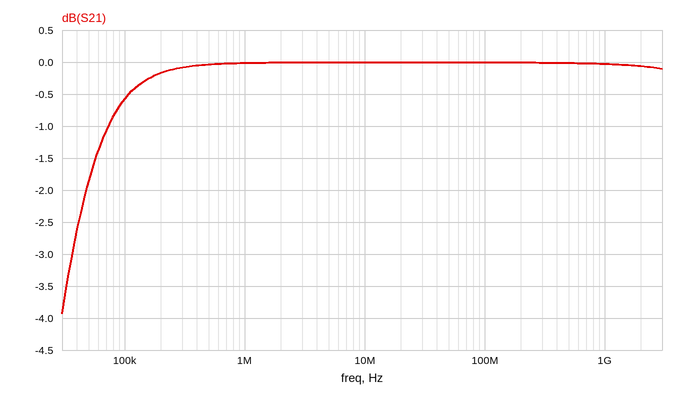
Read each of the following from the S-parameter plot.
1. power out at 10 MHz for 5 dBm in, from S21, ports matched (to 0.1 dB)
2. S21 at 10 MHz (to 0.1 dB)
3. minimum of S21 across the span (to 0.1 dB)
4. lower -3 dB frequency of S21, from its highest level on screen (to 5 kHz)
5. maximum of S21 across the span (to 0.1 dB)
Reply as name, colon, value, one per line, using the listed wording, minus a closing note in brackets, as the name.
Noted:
power out at 10 MHz for 5 dBm in, from S21, ports matched: 5.0 dBm
S21 at 10 MHz: 0.0 dB
minimum of S21 across the span: -3.9 dB
lower -3 dB frequency of S21, from its highest level on screen: 35 kHz
maximum of S21 across the span: 0.0 dB
